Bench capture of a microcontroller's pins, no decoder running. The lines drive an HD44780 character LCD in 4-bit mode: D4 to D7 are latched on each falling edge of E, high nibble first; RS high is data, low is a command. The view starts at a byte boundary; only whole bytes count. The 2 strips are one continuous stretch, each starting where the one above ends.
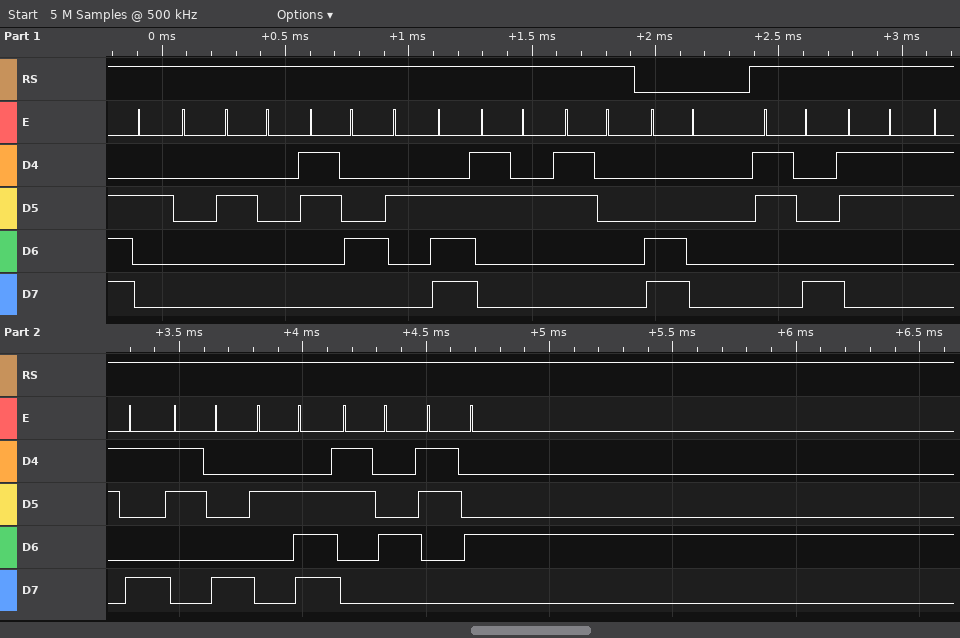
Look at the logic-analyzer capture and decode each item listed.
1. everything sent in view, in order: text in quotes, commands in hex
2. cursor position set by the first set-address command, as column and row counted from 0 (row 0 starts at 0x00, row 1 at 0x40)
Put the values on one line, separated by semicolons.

"  4.20" 0xC0 "8398.44"; column 0, row 1
